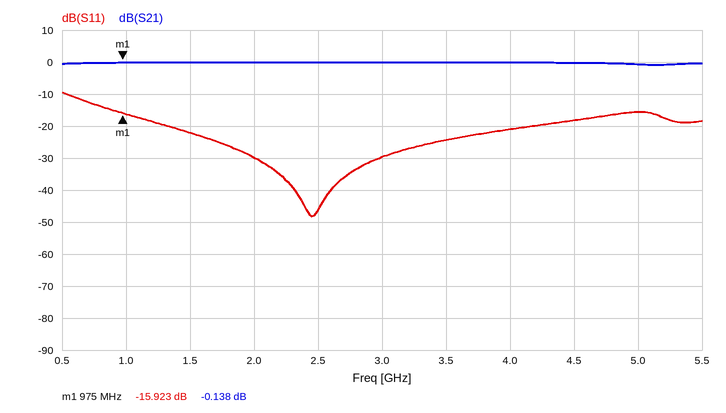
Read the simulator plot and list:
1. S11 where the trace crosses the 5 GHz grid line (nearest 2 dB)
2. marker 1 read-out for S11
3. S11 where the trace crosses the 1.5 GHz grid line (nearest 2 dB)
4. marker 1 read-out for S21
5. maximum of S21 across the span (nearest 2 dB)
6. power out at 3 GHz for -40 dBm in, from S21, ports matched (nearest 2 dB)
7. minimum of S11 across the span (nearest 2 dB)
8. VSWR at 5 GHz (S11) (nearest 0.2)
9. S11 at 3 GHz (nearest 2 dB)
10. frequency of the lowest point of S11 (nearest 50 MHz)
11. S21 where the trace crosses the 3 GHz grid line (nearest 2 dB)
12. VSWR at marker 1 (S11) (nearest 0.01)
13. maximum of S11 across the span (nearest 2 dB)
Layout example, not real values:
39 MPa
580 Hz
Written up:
-16 dB
-15.923 dB
-22 dB
-0.138 dB
0 dB
-40 dBm
-48 dB
1.4
-30 dB
2.45 GHz
0 dB
1.38
-10 dB
